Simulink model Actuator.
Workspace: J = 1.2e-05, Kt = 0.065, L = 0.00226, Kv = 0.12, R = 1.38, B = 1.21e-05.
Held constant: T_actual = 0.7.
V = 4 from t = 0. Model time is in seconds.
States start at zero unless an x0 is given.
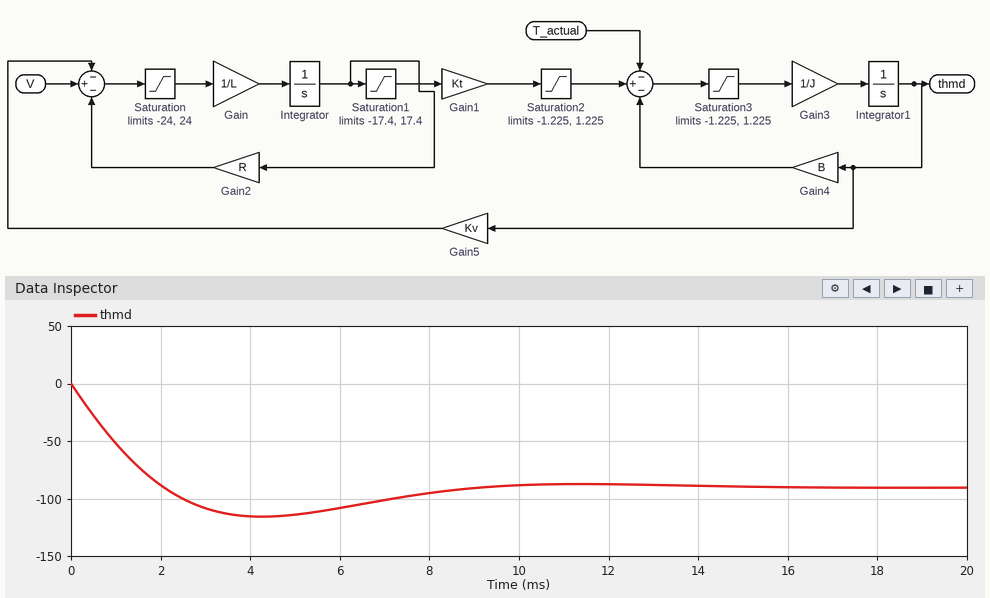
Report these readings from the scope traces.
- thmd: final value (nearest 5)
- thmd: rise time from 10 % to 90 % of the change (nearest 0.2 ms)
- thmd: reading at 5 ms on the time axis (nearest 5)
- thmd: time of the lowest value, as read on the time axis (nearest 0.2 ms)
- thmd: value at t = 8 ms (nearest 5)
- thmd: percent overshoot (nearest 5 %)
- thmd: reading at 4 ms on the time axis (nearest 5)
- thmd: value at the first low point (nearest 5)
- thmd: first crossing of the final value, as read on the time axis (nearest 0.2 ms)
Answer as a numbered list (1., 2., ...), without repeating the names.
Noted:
1. -90
2. 1.6 ms
3. -115
4. 4.2 ms
5. -95
6. 30 %
7. -115
8. -115
9. 2.0 ms
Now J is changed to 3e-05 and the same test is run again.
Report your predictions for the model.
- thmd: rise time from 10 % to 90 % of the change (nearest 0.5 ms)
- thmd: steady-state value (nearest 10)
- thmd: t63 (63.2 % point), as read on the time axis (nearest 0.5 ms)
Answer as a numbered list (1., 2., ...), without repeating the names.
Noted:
1. 6.5 ms
2. -90
3. 3.5 ms
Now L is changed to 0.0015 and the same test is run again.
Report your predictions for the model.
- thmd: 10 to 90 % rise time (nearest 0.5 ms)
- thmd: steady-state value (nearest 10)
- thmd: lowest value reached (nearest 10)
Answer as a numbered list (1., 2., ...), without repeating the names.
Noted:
1. 2.0 ms
2. -90
3. -100
